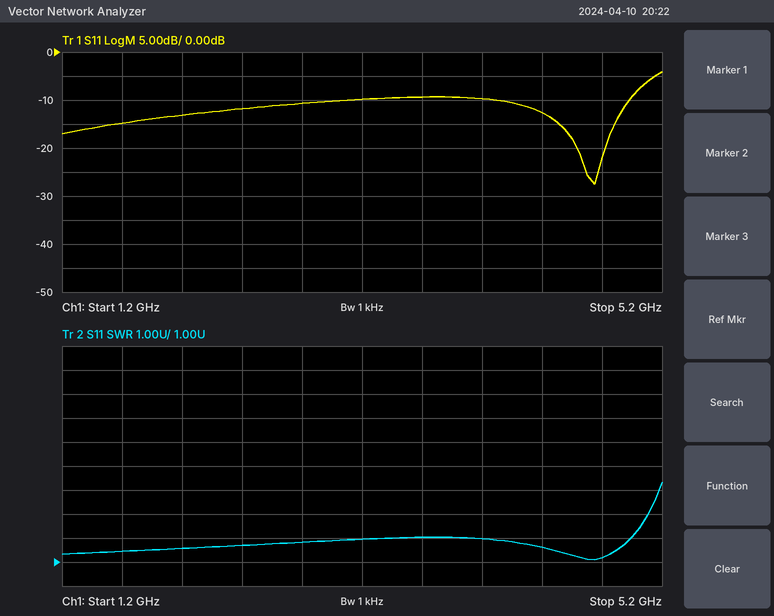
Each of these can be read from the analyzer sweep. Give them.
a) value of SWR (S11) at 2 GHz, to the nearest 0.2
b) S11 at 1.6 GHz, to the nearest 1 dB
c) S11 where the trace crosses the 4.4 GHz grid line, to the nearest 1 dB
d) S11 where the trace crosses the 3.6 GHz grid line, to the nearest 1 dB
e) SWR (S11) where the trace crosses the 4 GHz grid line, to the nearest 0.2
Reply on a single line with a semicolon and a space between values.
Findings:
1.6; -15 dB; -13 dB; -9 dB; 2.0
